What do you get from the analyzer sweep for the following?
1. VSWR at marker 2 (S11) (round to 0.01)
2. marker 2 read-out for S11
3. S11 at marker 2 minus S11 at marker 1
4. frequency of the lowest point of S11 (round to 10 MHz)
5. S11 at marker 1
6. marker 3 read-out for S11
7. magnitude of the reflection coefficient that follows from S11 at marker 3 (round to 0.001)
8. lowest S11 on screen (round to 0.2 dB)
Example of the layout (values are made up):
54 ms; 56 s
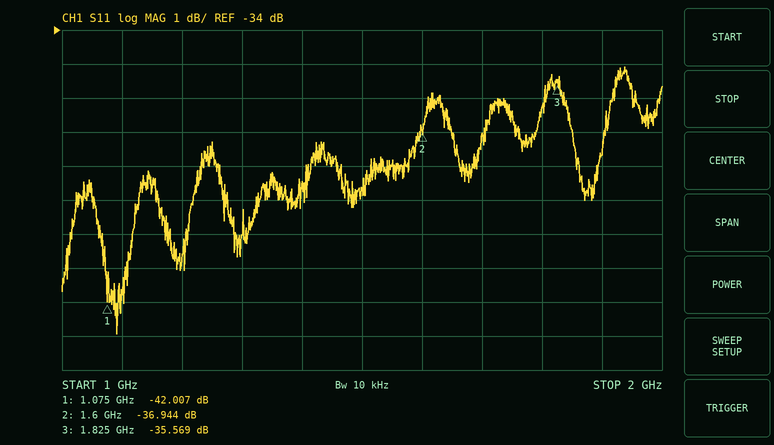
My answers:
1.03; -36.944 dB; 5.063 dB; 1.09 GHz; -42.007 dB; -35.569 dB; 0.017; -43.0 dB
